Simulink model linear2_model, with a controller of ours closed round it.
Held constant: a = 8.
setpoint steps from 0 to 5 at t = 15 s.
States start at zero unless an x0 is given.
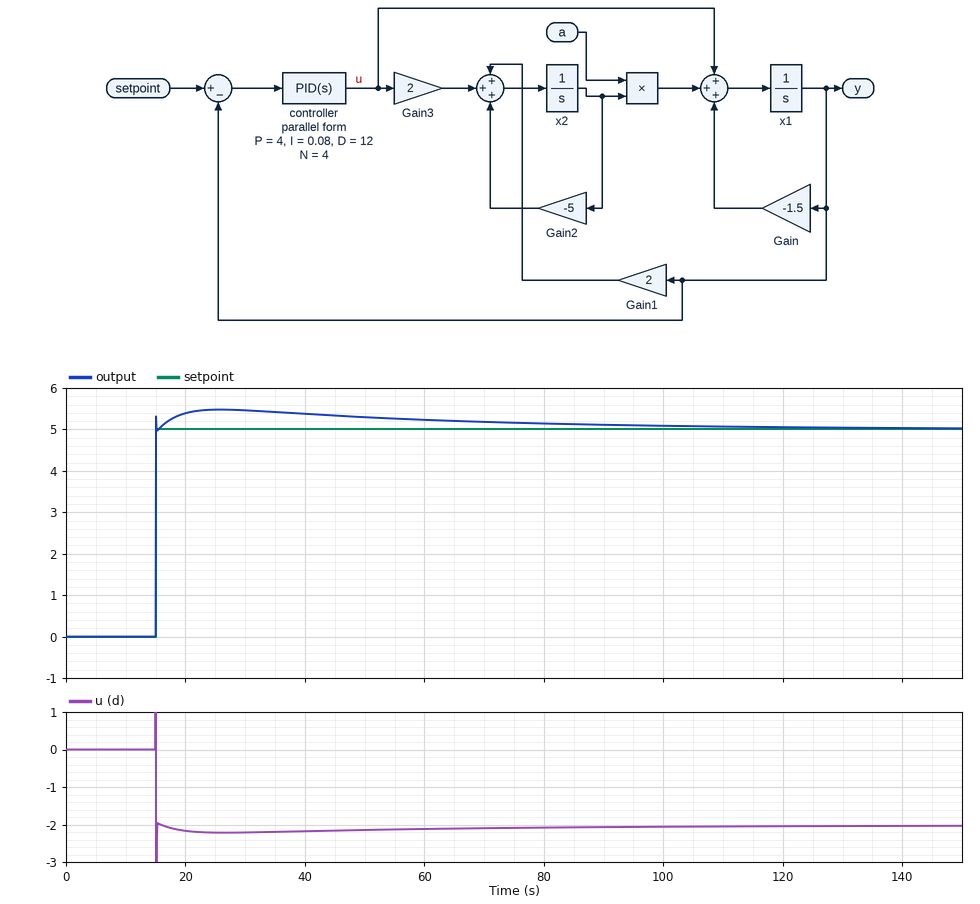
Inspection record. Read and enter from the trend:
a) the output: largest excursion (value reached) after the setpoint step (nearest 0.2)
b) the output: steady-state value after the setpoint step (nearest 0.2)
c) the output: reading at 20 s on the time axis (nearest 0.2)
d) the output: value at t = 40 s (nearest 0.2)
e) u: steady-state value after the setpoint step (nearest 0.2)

5.4
5.0
5.4
5.4
-2.0
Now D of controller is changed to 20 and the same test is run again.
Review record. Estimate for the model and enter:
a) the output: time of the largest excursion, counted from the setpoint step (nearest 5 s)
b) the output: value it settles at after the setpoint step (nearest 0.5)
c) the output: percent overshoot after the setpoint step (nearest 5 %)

15 s
5.0
10 %
